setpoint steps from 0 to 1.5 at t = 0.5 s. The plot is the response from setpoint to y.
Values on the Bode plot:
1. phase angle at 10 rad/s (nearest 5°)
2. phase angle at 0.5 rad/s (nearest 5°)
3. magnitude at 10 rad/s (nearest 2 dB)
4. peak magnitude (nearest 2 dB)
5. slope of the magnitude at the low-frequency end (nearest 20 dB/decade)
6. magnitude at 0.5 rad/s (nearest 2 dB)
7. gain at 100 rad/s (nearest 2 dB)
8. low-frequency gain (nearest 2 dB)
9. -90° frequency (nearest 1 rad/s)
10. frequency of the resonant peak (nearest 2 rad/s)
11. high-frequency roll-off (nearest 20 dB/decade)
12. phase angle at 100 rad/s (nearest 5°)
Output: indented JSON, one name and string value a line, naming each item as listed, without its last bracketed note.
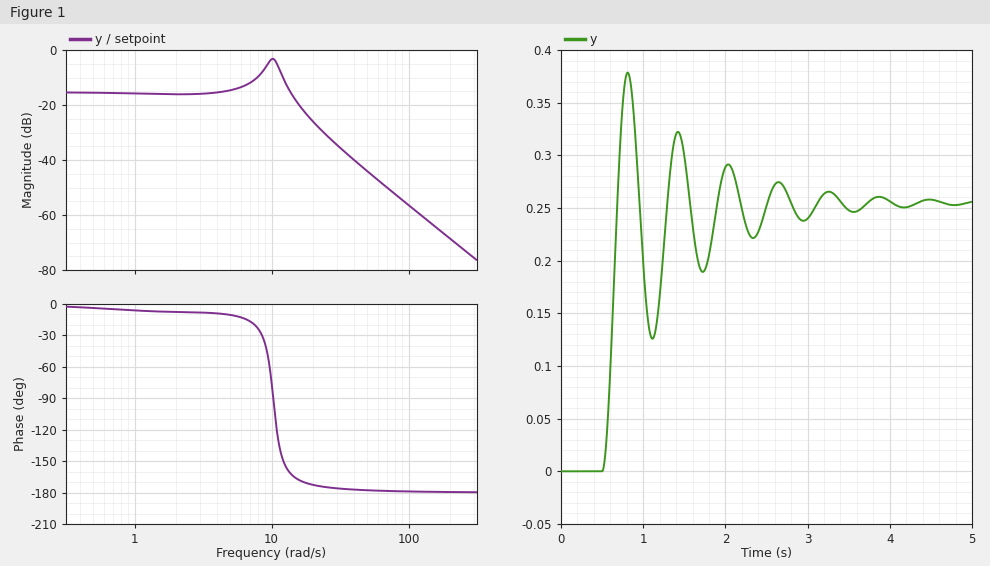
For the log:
{
  "phase angle at 10 rad/s": "-75°",
  "phase angle at 0.5 rad/s": "-5°",
  "magnitude at 10 rad/s": "-4 dB",
  "peak magnitude": "-4 dB",
  "slope of the magnitude at the low-frequency end": "0 dB/decade",
  "magnitude at 0.5 rad/s": "-16 dB",
  "gain at 100 rad/s": "-56 dB",
  "low-frequency gain": "-16 dB",
  "-90° frequency": "10 rad/s",
  "frequency of the resonant peak": "10 rad/s",
  "high-frequency roll-off": "-40 dB/decade",
  "phase angle at 100 rad/s": "-180°"
}
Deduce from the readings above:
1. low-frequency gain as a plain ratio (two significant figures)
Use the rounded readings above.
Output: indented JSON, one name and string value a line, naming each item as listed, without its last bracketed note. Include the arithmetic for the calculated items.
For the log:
{
  "low-frequency gain as a plain ratio": "10^(-16 / 20) = 0.16"
}
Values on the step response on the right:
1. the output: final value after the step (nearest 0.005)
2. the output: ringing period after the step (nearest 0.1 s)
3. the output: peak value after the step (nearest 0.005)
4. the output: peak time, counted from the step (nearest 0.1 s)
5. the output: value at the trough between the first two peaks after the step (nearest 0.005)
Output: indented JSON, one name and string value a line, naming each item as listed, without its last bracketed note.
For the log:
{
  "the output: final value after the step": "0.255",
  "the output: ringing period after the step": "0.6 s",
  "the output: peak value after the step": "0.380",
  "the output: peak time, counted from the step": "0.3 s",
  "the output: value at the trough between the first two peaks after the step": "0.125"
}
